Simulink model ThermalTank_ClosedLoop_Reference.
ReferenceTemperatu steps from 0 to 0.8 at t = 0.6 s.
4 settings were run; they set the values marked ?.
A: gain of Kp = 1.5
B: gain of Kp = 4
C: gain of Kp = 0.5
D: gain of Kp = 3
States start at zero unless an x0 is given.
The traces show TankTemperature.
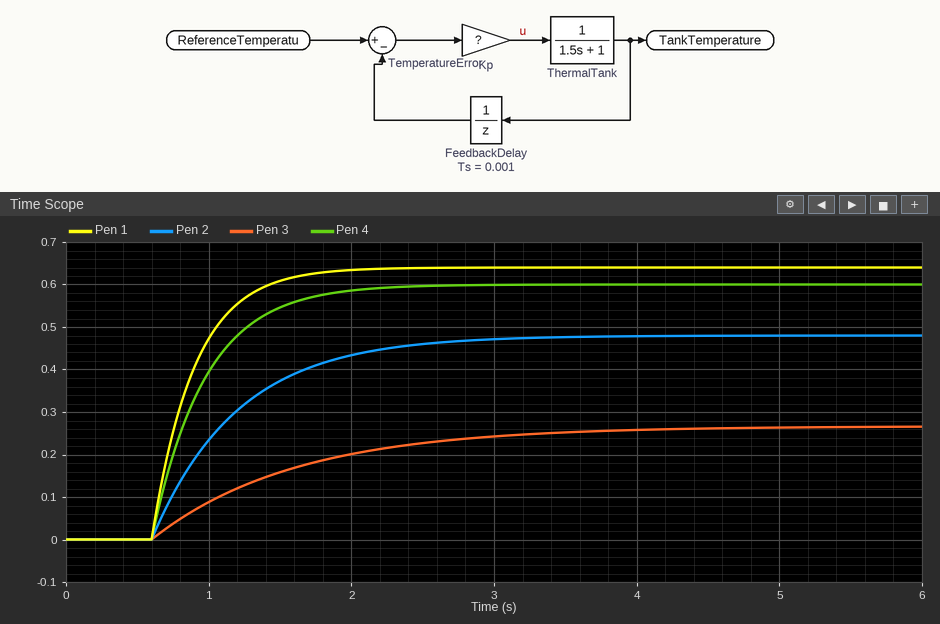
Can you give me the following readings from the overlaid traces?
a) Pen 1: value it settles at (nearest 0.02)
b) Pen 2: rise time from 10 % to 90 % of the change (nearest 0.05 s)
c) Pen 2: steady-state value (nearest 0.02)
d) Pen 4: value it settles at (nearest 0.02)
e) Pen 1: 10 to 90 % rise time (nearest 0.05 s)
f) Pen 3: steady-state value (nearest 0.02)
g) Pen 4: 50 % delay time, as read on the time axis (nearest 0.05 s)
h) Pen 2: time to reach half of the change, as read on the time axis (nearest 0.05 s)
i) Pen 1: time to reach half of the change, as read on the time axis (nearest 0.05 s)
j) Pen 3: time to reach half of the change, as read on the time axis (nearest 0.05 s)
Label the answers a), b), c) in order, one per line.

a) 0.64
b) 1.30 s
c) 0.48
d) 0.60
e) 0.65 s
f) 0.26
g) 0.85 s
h) 1.00 s
i) 0.80 s
j) 1.30 s
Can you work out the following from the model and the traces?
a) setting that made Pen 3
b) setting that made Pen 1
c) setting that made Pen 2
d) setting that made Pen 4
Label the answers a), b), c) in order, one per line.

a) C
b) B
c) A
d) D
